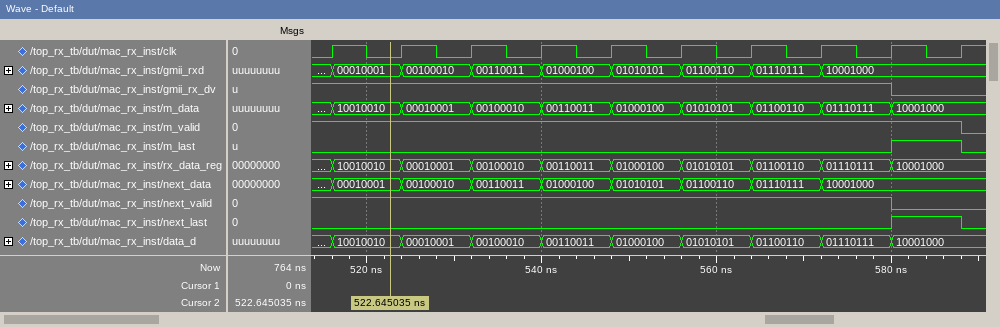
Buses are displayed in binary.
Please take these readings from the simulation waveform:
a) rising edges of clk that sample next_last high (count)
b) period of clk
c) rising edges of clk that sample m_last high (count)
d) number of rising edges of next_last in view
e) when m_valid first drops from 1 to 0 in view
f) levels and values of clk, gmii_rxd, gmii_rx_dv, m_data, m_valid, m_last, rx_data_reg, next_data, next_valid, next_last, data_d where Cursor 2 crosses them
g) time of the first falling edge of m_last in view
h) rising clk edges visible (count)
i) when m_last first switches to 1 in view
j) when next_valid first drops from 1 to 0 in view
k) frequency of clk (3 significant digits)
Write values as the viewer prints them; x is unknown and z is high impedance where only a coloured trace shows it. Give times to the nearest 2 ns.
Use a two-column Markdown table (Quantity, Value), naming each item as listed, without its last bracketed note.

| Quantity | Value |
|---|---|
| rising edges of clk that sample next_last high | 1 |
| period of clk | 8 ns |
| rising edges of clk that sample m_last high | 1 |
| number of rising edges of next_last in view | 1 |
| when m_valid first drops from 1 to 0 in view | 588 ns |
| levels and values of clk, gmii_rxd, gmii_rx_dv, m_data, m_valid, m_last, rx_data_reg, next_data, next_valid, next_last, data_d where Cursor 2 crosses them | clk=0, gmii_rxd=00010001, gmii_rx_dv=1, m_data=10010010, m_valid=1, m_last=0, rx_data_reg=10010010, next_data=00010001, next_valid=1, next_last=0, data_d=10010010 |
| time of the first falling edge of m_last in view | 588 ns |
| rising clk edges visible | 10 |
| when m_last first switches to 1 in view | 580 ns |
| when next_valid first drops from 1 to 0 in view | 580 ns |
| frequency of clk | 125 MHz |
